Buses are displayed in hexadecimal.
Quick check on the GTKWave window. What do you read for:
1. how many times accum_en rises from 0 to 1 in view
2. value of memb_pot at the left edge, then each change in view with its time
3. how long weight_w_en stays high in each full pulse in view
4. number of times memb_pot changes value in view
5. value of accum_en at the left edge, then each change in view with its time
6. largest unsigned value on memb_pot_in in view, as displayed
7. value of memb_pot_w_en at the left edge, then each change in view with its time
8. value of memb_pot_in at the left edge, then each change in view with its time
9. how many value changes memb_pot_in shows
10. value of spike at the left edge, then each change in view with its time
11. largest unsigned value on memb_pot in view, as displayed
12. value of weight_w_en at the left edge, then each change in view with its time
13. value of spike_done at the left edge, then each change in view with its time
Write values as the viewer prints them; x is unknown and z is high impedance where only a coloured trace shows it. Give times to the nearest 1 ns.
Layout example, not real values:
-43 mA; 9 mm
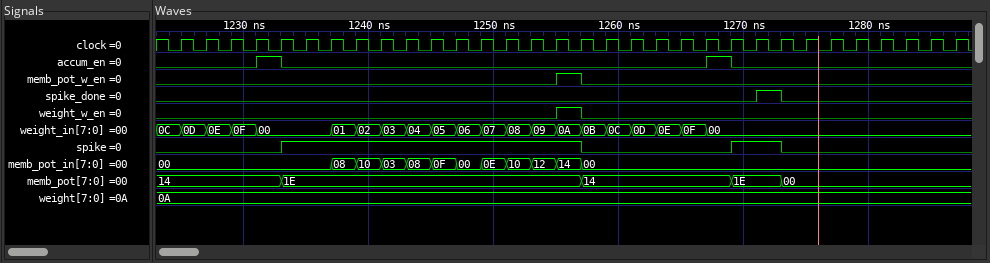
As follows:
2; 14, 1E at 1233 ns, 14 at 1257 ns, 1E at 1269 ns, 00 at 1273 ns; 2 ns; 4; 0, 1 at 1231 ns, 0 at 1233 ns, 1 at 1267 ns, 0 at 1269 ns; 14; 0, 1 at 1255 ns, 0 at 1257 ns; 00, 08 at 1237 ns, 10 at 1239 ns, 03 at 1241 ns, 08 at 1243 ns, 0F at 1245 ns, 00 at 1247 ns, 0E at 1249 ns, 10 at 1251 ns, 12 at 1253 ns, 14 at 1255 ns, 00 at 1257 ns; 11; 0, 1 at 1233 ns, 0 at 1257 ns, 1 at 1269 ns, 0 at 1273 ns; 1E; 0, 1 at 1255 ns, 0 at 1257 ns; 0, 1 at 1271 ns, 0 at 1273 ns
